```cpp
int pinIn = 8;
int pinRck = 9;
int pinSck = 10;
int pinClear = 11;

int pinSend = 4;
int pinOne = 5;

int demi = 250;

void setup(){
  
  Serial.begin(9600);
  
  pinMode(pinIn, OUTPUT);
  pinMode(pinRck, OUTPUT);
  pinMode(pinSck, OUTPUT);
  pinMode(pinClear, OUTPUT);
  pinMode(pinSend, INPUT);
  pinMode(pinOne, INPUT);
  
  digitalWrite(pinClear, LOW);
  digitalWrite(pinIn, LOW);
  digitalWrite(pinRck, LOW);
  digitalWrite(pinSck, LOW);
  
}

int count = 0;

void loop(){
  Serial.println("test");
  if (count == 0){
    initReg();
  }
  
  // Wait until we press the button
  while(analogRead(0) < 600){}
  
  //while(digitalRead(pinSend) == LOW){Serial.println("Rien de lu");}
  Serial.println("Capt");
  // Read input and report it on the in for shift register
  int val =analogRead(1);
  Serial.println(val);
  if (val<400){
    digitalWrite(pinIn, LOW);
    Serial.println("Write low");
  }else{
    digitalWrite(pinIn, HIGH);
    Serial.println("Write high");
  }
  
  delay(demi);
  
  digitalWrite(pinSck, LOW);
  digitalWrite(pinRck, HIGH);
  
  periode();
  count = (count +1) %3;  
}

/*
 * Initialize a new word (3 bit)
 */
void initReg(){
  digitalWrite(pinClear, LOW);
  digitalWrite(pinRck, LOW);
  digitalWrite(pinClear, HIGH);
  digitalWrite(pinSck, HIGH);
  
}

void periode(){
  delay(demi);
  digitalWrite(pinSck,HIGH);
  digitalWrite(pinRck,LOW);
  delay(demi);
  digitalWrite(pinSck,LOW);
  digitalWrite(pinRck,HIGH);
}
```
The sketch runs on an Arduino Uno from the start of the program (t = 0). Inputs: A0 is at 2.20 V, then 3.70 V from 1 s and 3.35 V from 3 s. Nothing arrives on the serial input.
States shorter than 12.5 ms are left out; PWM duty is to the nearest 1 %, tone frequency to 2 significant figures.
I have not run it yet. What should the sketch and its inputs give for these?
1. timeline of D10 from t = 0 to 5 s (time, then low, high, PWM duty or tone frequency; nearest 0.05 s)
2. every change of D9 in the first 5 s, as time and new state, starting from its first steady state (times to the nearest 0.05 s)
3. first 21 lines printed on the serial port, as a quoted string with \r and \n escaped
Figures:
0 s high; 1.25 s low; 1.5 s high; 1.75 s low; 2.25 s high; 2.5 s low; 3 s high; 3.5 s low; 3.75 s high; 4 s low; 4.5 s high; 4.75 s low
0 s low; 1.25 s high; 1.5 s low; 1.75 s high; 2.25 s low; 2.5 s high; 3 s low; 3.5 s high; 3.75 s low; 4 s high; 4.5 s low; 4.75 s high
"test\r\nCapt\r\n0\r\nWrite low\r\ntest\r\nCapt\r\n0\r\nWrite low\r\ntest\r\nCapt\r\n0\r\nWrite low\r\ntest\r\nCapt\r\n0\r\nWrite low\r\ntest\r\nCapt\r\n0\r\nWrite low\r\ntest\r\n"
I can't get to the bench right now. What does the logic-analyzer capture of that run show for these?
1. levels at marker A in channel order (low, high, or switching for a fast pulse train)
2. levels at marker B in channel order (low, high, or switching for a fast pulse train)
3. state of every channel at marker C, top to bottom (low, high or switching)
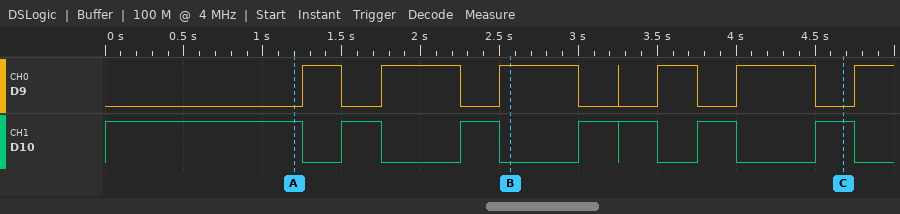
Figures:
D9 low, D10 high
D9 high, D10 low
D9 low, D10 high
